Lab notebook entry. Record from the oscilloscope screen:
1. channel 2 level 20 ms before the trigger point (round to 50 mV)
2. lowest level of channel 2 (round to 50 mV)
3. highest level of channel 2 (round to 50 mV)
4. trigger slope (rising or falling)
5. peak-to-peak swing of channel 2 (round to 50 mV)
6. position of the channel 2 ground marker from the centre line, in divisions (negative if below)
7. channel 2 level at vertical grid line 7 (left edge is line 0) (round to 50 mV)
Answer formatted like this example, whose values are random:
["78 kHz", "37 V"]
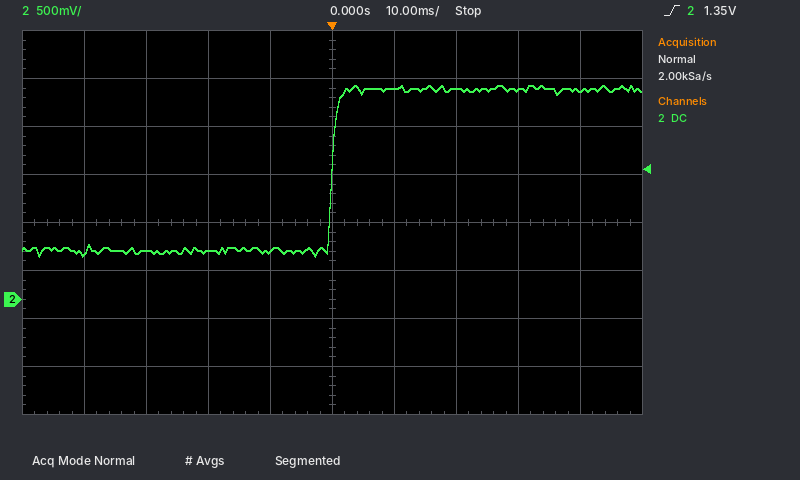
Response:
["500 mV", "450 mV", "2.25 V", "rising", "1.80 V", "-1.6 div", "2.20 V"]
